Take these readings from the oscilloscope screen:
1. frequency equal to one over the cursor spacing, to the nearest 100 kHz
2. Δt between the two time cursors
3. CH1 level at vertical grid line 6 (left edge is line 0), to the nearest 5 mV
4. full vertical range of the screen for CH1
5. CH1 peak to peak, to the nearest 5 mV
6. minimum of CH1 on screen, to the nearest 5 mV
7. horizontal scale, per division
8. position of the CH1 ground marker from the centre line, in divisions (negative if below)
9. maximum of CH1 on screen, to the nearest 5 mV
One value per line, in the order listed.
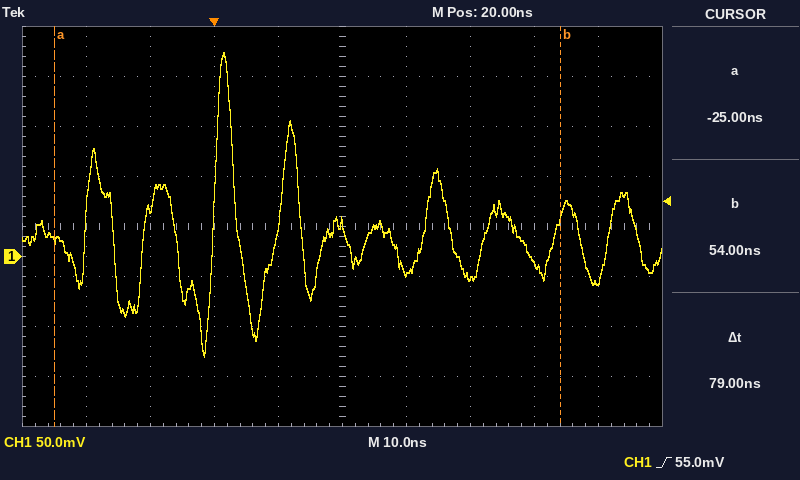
12.7 MHz
79 ns
-15 mV
400 mV
305 mV
-100 mV
10 ns
-0.6 div
205 mV
